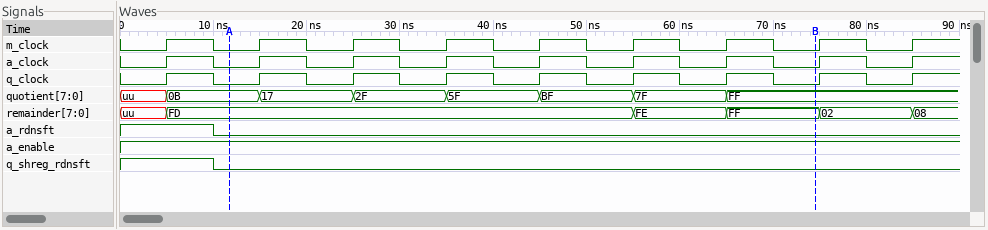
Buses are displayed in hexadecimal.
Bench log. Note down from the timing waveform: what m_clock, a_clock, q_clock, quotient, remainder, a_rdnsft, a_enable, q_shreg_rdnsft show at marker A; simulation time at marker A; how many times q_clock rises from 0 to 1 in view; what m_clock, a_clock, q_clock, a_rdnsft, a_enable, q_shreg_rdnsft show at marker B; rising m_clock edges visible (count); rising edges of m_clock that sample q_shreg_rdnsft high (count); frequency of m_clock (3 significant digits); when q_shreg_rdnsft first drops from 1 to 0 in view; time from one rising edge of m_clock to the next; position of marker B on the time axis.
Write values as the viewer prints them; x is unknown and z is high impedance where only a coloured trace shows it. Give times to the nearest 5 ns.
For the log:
m_clock=0, a_clock=0, q_clock=0, quotient=0B, remainder=FD, a_rdnsft=0, a_enable=1, q_shreg_rdnsft=0
10 ns
9
m_clock=0, a_clock=0, q_clock=0, a_rdnsft=0, a_enable=1, q_shreg_rdnsft=0
9
1
100 MHz
10 ns
10 ns
75 ns
